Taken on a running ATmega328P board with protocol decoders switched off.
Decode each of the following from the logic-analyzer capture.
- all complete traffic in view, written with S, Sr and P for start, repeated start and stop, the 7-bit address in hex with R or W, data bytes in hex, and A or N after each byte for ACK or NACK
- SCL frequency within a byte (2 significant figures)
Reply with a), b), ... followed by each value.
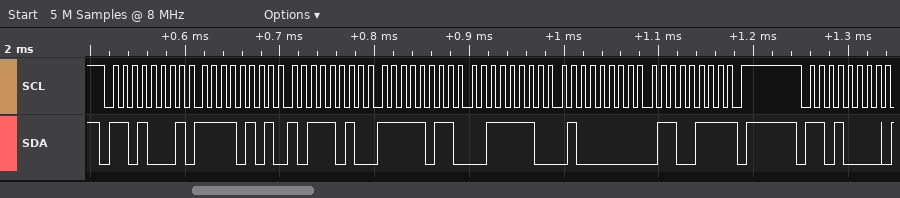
a) S 68R A F5 A BA A FB A 3E A 40 A 67 N P S 68W A
b) 100 kHz
